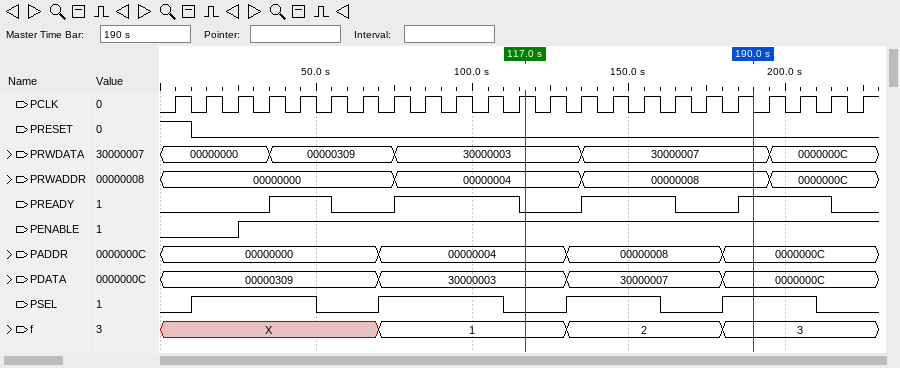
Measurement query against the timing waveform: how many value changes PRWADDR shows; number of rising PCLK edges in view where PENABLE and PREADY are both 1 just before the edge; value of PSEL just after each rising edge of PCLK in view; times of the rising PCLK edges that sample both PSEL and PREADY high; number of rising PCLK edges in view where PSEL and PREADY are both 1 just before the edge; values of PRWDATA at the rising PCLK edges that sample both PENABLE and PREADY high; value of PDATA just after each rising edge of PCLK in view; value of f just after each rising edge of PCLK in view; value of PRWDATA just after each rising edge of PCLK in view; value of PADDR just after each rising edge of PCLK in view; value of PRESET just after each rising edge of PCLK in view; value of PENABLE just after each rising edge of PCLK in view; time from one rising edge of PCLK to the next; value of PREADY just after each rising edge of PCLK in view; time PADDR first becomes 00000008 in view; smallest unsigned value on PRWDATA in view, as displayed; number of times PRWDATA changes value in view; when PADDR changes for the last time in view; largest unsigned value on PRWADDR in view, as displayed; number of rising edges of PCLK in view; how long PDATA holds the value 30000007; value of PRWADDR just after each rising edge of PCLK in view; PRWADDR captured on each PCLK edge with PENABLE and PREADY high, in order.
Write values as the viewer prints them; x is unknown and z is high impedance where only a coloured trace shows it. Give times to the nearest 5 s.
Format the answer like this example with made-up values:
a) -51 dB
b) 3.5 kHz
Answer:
a) 3
b) 12
c) 0 1 1 1 1 0 0 1 1 1 1 0 0 1 1 1 0 0 1 1 1 0 0
d) 45 s, 85 s, 95 s, 105 s, 145 s, 155 s, 195 s, 205 s
e) 8
f) 00000309, 00000309, 30000003, 30000003, 30000003, 30000003, 30000007, 30000007, 30000007, 30000007, 0000000C, 0000000C
g) 00000309, 00000309, 00000309, 00000309, 00000309, 00000309, 00000309, 30000003, 30000003, 30000003, 30000003, 30000003, 30000003, 30000007, 30000007, 30000007, 30000007, 30000007, 0000000C, 0000000C, 0000000C, 0000000C, 0000000C
h) X, X, X, X, X, X, X, 1, 1, 1, 1, 1, 1, 2, 2, 2, 2, 2, 3, 3, 3, 3, 3
i) 00000000, 00000000, 00000000, 00000309, 00000309, 00000309, 00000309, 30000003, 30000003, 30000003, 30000003, 30000003, 30000003, 30000007, 30000007, 30000007, 30000007, 30000007, 30000007, 0000000C, 0000000C, 0000000C, 0000000C
j) 00000000, 00000000, 00000000, 00000000, 00000000, 00000000, 00000000, 00000004, 00000004, 00000004, 00000004, 00000004, 00000004, 00000008, 00000008, 00000008, 00000008, 00000008, 0000000C, 0000000C, 0000000C, 0000000C, 0000000C
k) 1 0 0 0 0 0 0 0 0 0 0 0 0 0 0 0 0 0 0 0 0 0 0
l) 0 0 1 1 1 1 1 1 1 1 1 1 1 1 1 1 1 1 1 1 1 1 1
m) 10 s
n) 0 0 0 1 1 0 0 1 1 1 1 0 0 1 1 1 0 0 1 1 1 0 0
o) 130 s
p) 00000000
q) 4
r) 180 s
s) 0000000C
t) 23
u) 50 s
v) 00000000, 00000000, 00000000, 00000000, 00000000, 00000000, 00000000, 00000004, 00000004, 00000004, 00000004, 00000004, 00000004, 00000008, 00000008, 00000008, 00000008, 00000008, 00000008, 0000000C, 0000000C, 0000000C, 0000000C
w) 00000000, 00000000, 00000004, 00000004, 00000004, 00000004, 00000008, 00000008, 00000008, 00000008, 0000000C, 0000000C
